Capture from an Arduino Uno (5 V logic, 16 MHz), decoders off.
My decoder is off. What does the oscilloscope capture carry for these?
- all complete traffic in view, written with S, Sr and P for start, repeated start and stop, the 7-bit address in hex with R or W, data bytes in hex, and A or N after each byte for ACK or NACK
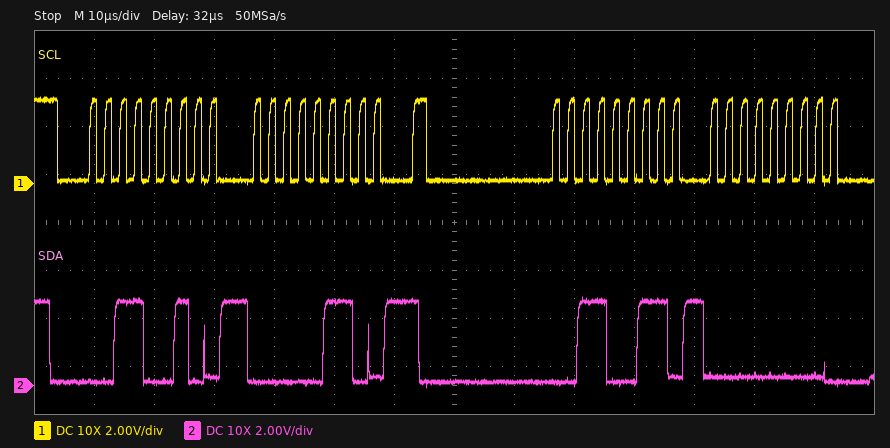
S 19W A 06 A Sr 19R A 00 A
